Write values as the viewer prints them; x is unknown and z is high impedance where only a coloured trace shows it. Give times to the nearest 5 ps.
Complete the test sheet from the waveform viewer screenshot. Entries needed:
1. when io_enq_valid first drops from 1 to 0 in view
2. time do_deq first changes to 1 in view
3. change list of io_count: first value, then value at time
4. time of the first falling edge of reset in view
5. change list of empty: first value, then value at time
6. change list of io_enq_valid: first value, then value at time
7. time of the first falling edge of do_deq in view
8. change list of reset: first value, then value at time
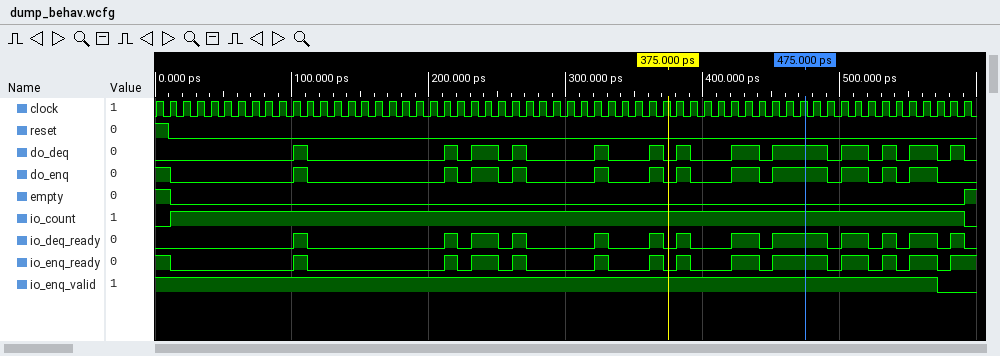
570 ps
100 ps
0, 1 at 10 ps, 0 at 590 ps
10 ps
1, 0 at 10 ps, 1 at 590 ps
1, 0 at 570 ps
110 ps
1, 0 at 10 ps
